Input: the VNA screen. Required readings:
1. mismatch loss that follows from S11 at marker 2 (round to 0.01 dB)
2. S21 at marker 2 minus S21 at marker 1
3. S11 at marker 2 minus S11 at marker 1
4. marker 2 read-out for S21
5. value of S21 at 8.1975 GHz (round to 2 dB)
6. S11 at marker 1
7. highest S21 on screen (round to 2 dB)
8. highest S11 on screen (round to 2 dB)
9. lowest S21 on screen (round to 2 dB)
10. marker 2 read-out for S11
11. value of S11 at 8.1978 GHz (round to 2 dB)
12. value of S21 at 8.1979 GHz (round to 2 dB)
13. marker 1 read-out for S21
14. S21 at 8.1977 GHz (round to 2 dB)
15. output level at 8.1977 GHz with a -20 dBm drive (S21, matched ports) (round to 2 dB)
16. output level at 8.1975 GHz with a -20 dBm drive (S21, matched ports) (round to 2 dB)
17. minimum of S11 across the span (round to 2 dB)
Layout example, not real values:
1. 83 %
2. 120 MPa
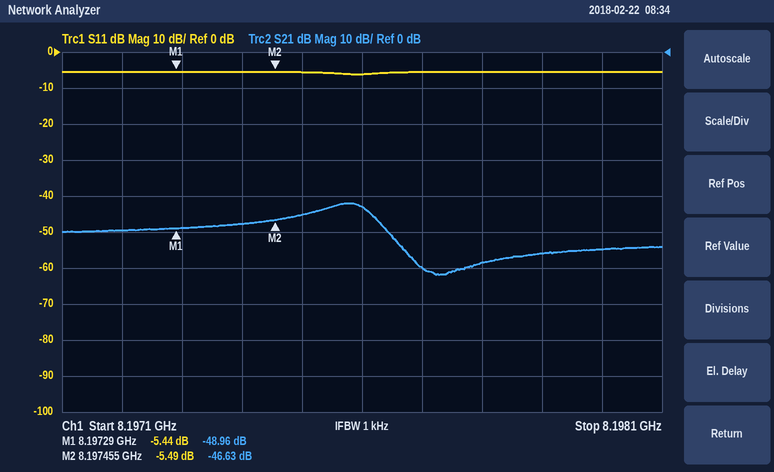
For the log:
1. 1.44 dB
2. 2.33 dB
3. -0.05 dB
4. -46.63 dB
5. -46 dB
6. -5.44 dB
7. -42 dB
8. -6 dB
9. -62 dB
10. -5.49 dB
11. -6 dB
12. -56 dB
13. -48.96 dB
14. -60 dB
15. -80 dBm
16. -66 dBm
17. -6 dB
